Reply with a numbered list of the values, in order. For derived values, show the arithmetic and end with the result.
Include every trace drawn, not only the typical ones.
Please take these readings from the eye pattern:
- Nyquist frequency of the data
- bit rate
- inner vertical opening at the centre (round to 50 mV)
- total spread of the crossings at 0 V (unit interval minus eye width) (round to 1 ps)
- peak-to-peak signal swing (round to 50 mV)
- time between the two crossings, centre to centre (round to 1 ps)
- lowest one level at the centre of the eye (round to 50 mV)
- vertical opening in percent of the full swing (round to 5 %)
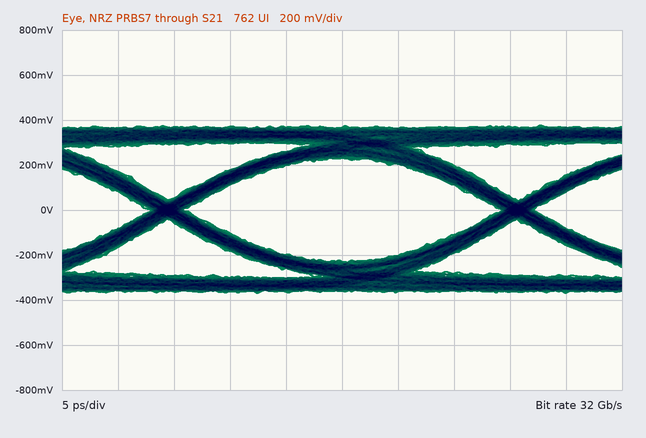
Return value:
1. 16 GHz
2. 32 Gb/s
3. 450 mV
4. 3 ps
5. 750 mV
6. 31 ps
7. 250 mV
8. 450 mV / 750 mV ≈ 60 %
